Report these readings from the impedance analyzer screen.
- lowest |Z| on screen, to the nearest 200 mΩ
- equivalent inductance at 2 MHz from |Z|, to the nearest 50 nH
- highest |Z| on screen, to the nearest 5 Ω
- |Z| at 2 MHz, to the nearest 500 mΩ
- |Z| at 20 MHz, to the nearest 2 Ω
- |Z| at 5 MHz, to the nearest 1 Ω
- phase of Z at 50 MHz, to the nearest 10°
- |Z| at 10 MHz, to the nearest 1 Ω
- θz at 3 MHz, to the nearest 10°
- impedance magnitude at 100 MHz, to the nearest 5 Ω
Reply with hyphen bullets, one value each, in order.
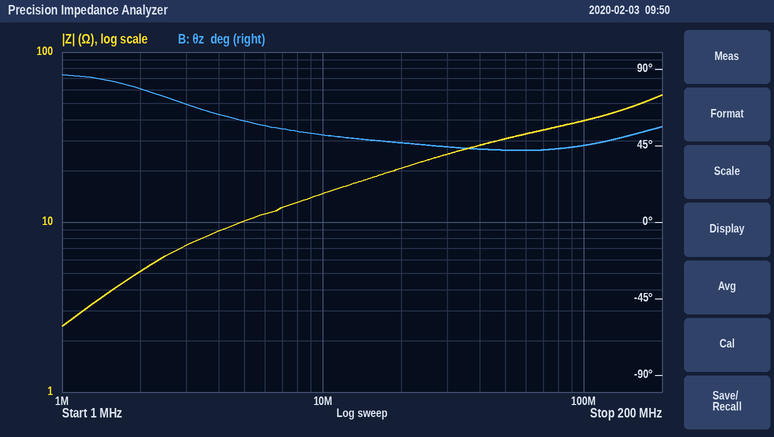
- 2.4 Ω
- 400 nH
- 55 Ω
- 5.0 Ω
- 20 Ω
- 10 Ω
- 40°
- 15 Ω
- 70°
- 40 Ω
